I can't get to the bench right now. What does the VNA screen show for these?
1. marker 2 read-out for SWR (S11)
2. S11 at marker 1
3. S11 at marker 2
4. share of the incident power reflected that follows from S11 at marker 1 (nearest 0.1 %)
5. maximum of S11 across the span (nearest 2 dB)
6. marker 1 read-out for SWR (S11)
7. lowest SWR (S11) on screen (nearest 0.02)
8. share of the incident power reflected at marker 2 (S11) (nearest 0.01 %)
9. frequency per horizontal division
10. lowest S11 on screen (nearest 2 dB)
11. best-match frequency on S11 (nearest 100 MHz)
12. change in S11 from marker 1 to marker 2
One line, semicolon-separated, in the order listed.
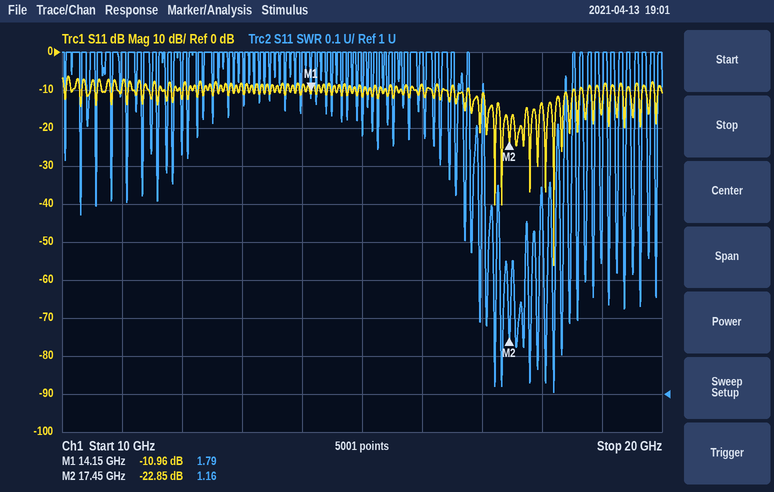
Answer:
1.16; -10.96 dB; -22.85 dB; 8.0 %; -6 dB; 1.79; 1.00; 0.52 %; 1 GHz; -56 dB; 18.2 GHz; -11.89 dB
